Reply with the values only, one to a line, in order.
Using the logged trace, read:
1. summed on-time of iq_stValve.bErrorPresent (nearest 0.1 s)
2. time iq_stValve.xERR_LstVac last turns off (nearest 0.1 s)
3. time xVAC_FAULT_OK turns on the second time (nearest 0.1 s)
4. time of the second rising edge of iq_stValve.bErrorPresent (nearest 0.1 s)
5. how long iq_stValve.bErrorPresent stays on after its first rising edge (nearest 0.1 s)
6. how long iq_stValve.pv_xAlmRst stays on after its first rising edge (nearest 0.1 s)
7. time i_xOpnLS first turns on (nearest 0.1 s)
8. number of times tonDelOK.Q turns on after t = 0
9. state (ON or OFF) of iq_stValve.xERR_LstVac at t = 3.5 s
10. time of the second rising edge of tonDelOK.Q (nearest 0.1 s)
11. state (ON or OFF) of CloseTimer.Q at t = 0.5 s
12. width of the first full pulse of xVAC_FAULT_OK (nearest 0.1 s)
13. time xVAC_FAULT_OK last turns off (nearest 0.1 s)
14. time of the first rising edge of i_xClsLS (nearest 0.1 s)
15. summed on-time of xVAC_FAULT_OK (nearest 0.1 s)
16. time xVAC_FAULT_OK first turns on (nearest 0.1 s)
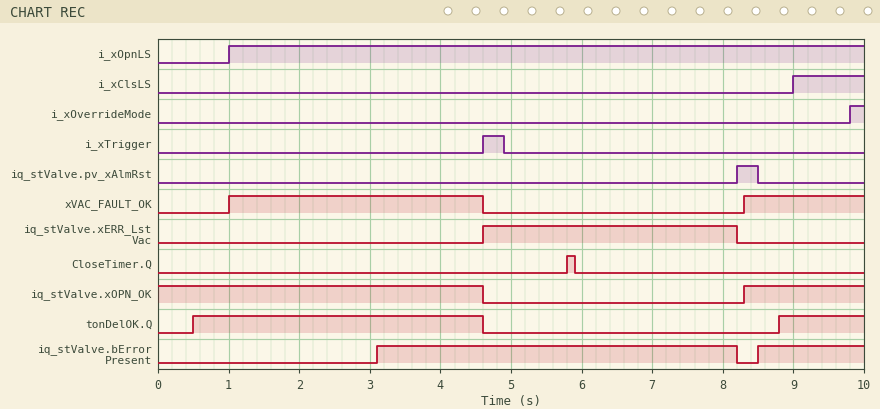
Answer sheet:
6.6 s
8.2 s
8.3 s
8.5 s
5.1 s
0.3 s
1.0 s
2
OFF
8.8 s
OFF
3.6 s
4.6 s
9.0 s
5.3 s
1.0 s
